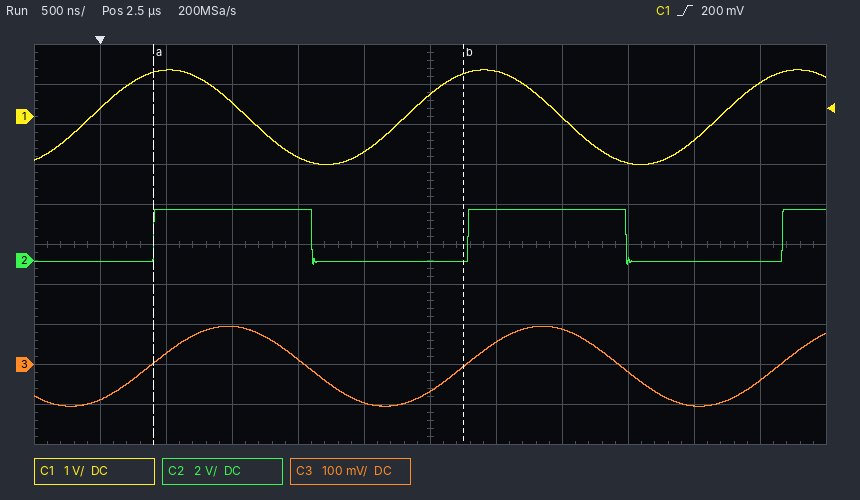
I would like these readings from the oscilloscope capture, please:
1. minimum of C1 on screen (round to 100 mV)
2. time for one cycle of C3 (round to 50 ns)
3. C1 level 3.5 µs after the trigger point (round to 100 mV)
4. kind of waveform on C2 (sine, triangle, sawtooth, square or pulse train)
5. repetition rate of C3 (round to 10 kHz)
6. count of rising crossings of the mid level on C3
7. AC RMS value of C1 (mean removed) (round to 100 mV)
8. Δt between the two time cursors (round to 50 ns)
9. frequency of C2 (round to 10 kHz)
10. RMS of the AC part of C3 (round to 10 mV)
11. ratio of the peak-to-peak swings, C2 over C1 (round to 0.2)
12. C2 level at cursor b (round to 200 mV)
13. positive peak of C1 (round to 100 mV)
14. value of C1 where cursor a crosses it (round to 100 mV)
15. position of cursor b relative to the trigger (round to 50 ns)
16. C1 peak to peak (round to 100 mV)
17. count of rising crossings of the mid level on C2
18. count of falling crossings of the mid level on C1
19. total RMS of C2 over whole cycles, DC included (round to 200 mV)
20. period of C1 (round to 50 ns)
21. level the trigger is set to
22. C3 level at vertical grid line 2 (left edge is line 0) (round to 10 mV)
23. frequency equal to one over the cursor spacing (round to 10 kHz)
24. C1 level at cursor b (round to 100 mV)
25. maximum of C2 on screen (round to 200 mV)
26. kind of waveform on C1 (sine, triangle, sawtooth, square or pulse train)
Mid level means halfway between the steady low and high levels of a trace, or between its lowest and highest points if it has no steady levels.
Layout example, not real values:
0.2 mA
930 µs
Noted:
-1.2 V
2.40 µs
0.0 V
square
420 kHz
3
800 mV
2.35 µs
420 kHz
70 mV
1.2
0.0 V
1.2 V
1.1 V
+2.75 µs
2.4 V
3
2
1.8 V
2.40 µs
200 mV
30 mV
430 kHz
1.1 V
2.6 V
sine
